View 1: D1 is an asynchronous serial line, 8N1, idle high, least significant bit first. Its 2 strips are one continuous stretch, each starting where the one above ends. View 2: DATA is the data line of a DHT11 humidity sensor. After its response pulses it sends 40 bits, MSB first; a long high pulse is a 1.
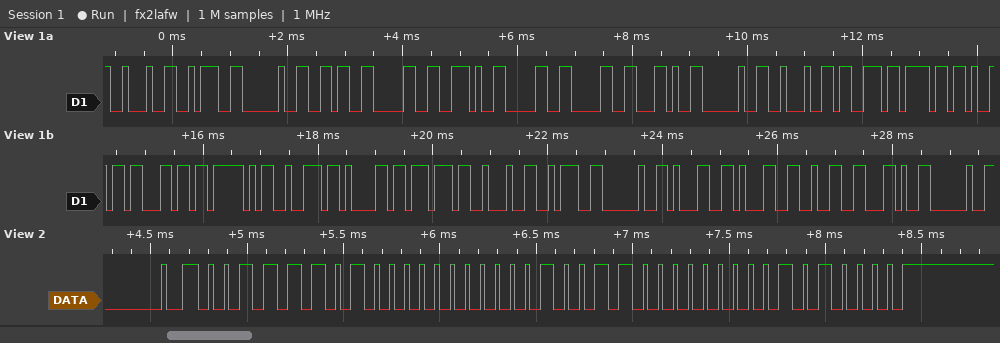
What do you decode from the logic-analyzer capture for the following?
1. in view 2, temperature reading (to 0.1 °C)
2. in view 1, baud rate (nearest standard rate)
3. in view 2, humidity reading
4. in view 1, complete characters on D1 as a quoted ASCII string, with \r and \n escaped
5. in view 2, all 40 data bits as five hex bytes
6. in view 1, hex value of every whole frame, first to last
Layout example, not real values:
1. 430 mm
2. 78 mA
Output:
1. 19.0 °C
2. 9600 baud
3. 61 %
4. "\": 60.00, \"soil_raw\": 112, "
5. 3D 00 13 00 50
6. 22 3A 20 36 30 2E 30 30 2C 20 22 73 6F 69 6C 5F 72 61 77 22 3A 20 31 31 32 2C 20
